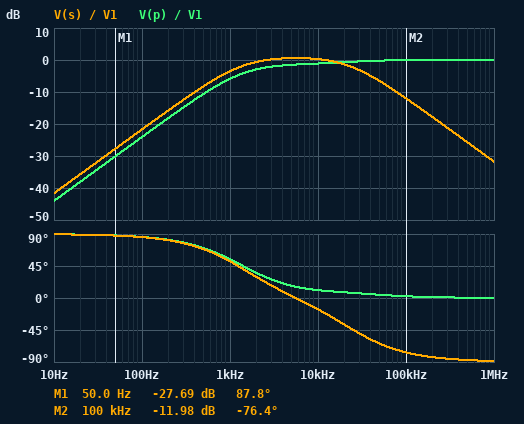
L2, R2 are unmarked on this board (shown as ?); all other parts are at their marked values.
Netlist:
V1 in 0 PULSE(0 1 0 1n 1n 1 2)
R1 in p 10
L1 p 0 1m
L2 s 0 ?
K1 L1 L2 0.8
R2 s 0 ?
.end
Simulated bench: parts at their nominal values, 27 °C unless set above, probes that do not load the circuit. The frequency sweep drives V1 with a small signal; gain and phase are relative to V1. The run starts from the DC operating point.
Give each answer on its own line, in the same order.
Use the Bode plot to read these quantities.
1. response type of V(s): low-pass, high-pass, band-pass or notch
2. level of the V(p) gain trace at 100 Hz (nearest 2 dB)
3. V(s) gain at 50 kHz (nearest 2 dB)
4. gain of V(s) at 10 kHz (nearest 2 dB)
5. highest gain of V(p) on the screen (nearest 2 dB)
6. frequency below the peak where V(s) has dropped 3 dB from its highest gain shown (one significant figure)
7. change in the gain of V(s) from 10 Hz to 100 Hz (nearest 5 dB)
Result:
band-pass
-24 dB
-6 dB
0 dB
0 dB
1 kHz
20 dB
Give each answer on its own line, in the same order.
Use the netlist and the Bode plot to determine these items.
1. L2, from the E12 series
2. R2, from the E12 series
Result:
2.7 mH
120 Ω
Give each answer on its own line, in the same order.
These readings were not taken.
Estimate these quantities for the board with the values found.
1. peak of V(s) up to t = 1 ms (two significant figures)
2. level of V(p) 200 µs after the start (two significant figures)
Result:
950 mV
150 mV
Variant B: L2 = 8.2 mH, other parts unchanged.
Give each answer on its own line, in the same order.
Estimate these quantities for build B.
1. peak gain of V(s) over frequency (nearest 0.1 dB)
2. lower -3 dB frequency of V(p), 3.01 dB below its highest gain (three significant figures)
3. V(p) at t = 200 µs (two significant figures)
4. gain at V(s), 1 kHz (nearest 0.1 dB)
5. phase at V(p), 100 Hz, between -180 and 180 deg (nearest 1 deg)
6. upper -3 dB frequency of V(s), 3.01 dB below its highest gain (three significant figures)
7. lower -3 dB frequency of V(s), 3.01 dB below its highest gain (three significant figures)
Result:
2.7 dB
4.44 kHz
170 mV
0.3 dB
85 deg
11.8 kHz
875 Hz
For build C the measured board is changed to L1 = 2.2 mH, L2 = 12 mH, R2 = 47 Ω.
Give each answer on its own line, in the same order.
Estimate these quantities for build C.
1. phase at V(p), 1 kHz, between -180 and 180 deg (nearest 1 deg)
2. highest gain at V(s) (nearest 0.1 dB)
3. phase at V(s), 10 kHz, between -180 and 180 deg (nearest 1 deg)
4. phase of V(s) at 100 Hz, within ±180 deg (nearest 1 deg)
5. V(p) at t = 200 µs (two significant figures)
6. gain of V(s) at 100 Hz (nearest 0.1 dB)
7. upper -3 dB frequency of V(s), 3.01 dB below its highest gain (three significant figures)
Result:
34 deg
-1.3 dB
-69 deg
73 deg
290 mV
-12.1 dB
4.05 kHz
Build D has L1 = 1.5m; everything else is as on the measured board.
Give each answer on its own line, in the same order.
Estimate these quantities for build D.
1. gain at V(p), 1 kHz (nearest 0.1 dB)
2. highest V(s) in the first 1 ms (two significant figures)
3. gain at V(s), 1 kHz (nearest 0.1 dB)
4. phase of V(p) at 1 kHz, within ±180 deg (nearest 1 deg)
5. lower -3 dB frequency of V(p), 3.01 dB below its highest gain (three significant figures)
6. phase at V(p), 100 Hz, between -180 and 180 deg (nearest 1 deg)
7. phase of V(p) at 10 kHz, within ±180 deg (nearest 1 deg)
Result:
-3.7 dB
840 mV
-3.1 dB
44 deg
1.19 kHz
84 deg
8 deg
